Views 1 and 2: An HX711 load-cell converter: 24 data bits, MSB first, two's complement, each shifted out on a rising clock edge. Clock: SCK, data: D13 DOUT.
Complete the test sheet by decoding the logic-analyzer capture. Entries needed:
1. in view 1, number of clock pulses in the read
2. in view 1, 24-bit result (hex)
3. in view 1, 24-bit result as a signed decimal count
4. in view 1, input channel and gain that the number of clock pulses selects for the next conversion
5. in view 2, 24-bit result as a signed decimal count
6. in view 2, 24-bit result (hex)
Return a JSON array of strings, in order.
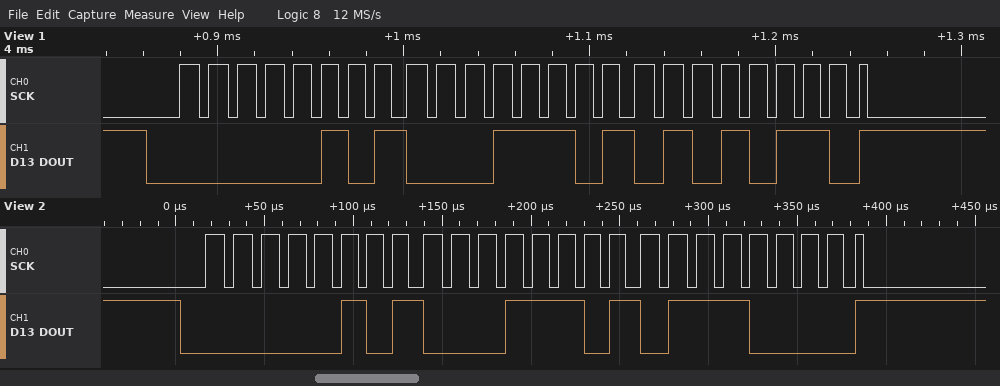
["25", "0x051D56", "335190", "channel A, gain 128", "335216", "0x051D70"]
